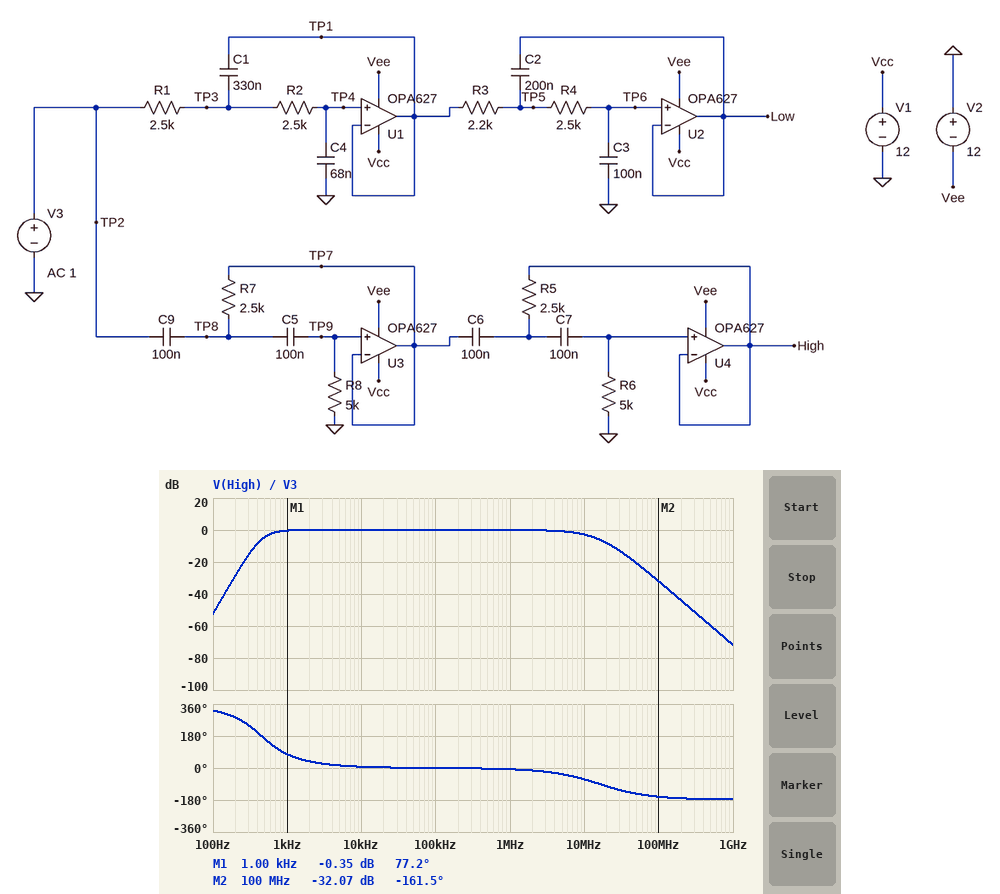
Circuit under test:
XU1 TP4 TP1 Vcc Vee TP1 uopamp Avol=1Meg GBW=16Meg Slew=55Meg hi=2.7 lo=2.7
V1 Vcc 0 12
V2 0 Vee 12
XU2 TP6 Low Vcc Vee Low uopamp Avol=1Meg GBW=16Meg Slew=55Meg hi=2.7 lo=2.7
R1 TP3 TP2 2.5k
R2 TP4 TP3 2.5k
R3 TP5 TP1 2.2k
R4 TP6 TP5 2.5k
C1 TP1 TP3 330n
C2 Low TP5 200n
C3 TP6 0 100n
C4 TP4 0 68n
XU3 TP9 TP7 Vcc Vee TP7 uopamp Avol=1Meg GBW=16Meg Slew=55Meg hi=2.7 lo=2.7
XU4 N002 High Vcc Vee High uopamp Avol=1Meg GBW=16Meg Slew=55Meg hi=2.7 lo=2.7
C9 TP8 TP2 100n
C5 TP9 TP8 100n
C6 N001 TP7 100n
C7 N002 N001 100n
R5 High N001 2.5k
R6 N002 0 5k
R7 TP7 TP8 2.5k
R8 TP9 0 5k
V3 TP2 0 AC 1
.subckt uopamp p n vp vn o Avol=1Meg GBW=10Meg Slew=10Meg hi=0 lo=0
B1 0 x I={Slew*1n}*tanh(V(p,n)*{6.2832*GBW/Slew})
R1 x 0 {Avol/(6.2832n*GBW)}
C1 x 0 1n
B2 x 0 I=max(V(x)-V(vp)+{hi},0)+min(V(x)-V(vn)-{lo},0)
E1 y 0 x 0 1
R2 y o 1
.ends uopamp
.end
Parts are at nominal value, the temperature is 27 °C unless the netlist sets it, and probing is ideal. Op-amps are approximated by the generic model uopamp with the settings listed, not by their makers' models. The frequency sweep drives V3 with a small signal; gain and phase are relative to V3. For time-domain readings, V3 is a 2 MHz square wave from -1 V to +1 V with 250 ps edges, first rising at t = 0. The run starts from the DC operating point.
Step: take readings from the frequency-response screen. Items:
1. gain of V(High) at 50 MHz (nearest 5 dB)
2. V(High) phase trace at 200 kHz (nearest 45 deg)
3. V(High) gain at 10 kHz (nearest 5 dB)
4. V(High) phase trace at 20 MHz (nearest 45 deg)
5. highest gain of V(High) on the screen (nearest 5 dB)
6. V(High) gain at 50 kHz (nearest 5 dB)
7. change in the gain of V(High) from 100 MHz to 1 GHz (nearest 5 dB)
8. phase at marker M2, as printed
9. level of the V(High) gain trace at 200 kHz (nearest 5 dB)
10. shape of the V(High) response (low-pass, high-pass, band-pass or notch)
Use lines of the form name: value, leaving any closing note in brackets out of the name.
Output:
gain of V(High) at 50 MHz: -20 dB
V(High) phase trace at 200 kHz: 0 deg
V(High) gain at 10 kHz: 0 dB
V(High) phase trace at 20 MHz: -90 deg
highest gain of V(High) on the screen: 0 dB
V(High) gain at 50 kHz: 0 dB
change in the gain of V(High) from 100 MHz to 1 GHz: -40 dB
phase at marker M2, as printed: -161.5 deg
level of the V(High) gain trace at 200 kHz: 0 dB
shape of the V(High) response: band-pass
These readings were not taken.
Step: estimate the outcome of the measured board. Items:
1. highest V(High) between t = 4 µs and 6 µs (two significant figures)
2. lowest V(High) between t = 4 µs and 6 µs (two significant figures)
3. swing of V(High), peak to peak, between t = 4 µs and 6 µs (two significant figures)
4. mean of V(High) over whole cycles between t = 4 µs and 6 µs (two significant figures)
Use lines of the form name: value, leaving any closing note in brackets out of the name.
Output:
highest V(High) between t = 4 µs and 6 µs: 2.0 V
lowest V(High) between t = 4 µs and 6 µs: -47 mV
swing of V(High), peak to peak, between t = 4 µs and 6 µs: 2.0 V
mean of V(High) over whole cycles between t = 4 µs and 6 µs: 960 mV
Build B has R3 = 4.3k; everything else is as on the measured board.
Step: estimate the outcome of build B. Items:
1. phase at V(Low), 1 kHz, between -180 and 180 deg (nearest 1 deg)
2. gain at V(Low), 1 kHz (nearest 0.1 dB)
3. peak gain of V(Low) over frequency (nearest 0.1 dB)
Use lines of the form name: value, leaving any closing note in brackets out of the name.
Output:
phase at V(Low), 1 kHz, between -180 and 180 deg: 55 deg
gain at V(Low), 1 kHz: -32.7 dB
peak gain of V(Low) over frequency: 0.4 dB
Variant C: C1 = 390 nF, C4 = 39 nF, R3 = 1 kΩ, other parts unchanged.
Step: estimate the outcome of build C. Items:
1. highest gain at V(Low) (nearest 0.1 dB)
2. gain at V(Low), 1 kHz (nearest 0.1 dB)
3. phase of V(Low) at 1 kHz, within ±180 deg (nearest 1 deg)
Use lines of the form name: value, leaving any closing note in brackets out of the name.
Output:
highest gain at V(Low): 3.2 dB
gain at V(Low), 1 kHz: -17.2 dB
phase of V(Low) at 1 kHz, within ±180 deg: 90 deg
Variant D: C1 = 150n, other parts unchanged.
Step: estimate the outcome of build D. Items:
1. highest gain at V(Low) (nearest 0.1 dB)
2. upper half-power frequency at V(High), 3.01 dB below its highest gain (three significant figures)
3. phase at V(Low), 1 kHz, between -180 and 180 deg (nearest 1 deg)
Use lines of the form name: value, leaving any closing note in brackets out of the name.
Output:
highest gain at V(Low): 0 dB
upper half-power frequency at V(High), 3.01 dB below its highest gain: 10.3 MHz
phase at V(Low), 1 kHz, between -180 and 180 deg: 96 deg
